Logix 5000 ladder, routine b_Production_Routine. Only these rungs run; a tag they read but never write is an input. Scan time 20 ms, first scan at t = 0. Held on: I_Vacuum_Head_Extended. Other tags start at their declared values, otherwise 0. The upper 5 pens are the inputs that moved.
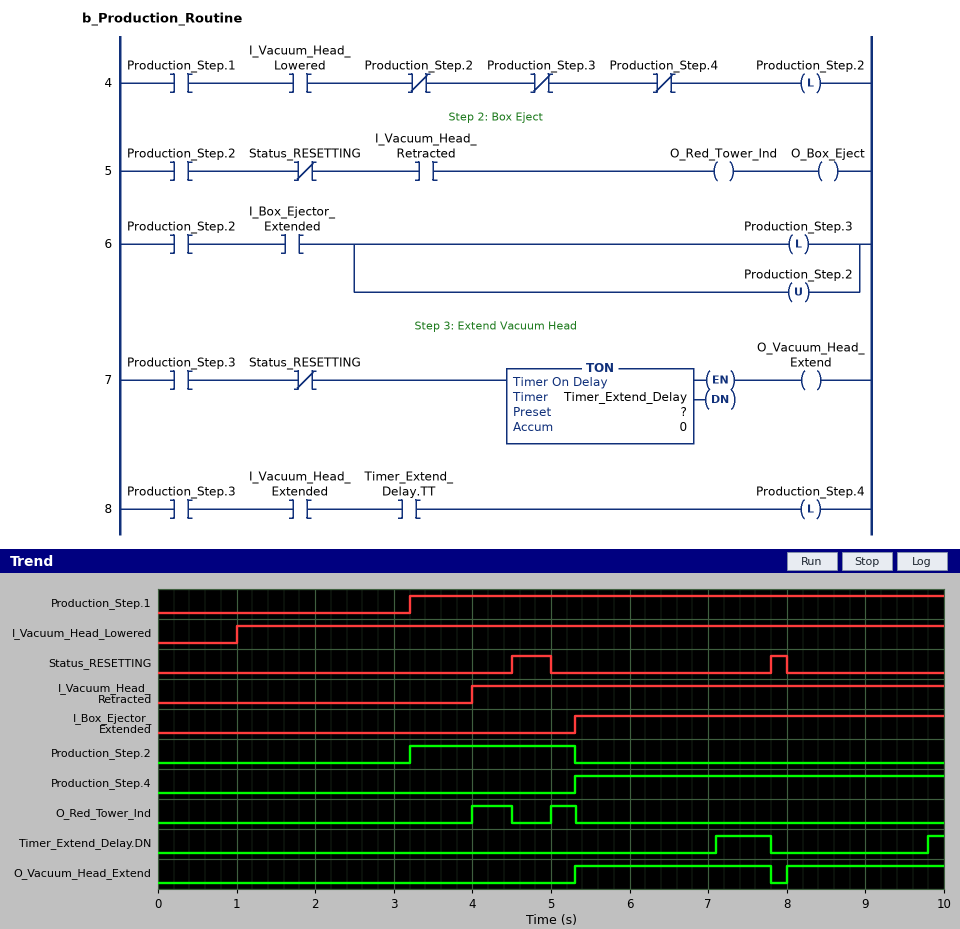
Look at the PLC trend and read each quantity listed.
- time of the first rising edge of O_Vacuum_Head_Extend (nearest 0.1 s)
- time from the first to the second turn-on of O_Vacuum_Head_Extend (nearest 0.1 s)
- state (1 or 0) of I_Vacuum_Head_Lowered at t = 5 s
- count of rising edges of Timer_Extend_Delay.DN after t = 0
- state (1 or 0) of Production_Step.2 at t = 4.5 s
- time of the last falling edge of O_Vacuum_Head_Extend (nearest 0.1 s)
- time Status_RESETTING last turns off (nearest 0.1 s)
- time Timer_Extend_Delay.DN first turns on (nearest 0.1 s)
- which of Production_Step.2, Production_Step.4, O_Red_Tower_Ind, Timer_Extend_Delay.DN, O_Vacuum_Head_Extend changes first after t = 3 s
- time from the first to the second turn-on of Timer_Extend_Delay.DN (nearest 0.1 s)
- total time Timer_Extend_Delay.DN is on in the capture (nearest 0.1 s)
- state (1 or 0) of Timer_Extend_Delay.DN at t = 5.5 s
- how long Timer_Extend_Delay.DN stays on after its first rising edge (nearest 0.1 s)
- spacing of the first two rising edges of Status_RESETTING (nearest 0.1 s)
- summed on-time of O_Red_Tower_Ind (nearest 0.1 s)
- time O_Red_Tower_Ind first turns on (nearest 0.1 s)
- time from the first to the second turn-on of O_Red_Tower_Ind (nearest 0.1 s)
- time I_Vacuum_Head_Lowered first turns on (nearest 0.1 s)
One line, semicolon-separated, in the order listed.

5.3 s; 2.7 s; 1; 2; 1; 7.8 s; 8.0 s; 7.1 s; Production_Step.2; 2.7 s; 0.9 s; 0; 0.7 s; 3.3 s; 0.8 s; 4.0 s; 1.0 s; 1.0 s
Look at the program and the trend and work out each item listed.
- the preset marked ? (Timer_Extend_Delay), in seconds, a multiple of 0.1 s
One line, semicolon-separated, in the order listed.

1.8 s
